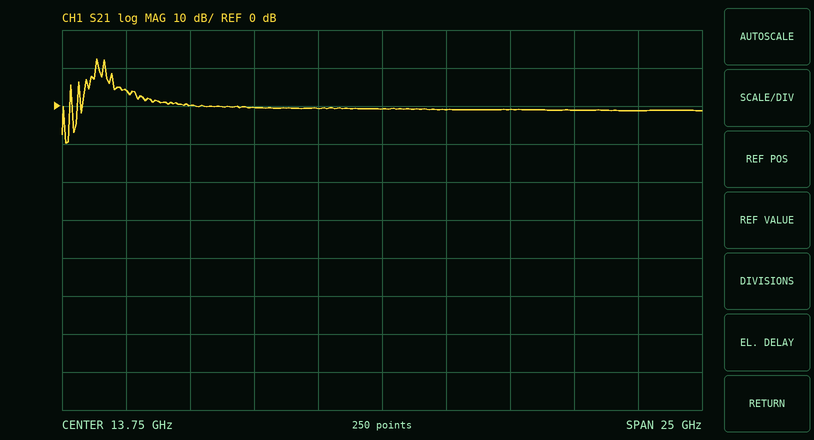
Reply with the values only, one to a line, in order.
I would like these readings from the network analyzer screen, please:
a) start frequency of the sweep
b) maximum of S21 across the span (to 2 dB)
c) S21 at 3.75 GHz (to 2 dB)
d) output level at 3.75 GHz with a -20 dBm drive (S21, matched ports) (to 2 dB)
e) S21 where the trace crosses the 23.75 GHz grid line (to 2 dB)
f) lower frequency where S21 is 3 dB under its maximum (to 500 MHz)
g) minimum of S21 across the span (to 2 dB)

1.25 GHz
12 dB
4 dB
-16 dBm
-2 dB
2.5 GHz
-10 dB
